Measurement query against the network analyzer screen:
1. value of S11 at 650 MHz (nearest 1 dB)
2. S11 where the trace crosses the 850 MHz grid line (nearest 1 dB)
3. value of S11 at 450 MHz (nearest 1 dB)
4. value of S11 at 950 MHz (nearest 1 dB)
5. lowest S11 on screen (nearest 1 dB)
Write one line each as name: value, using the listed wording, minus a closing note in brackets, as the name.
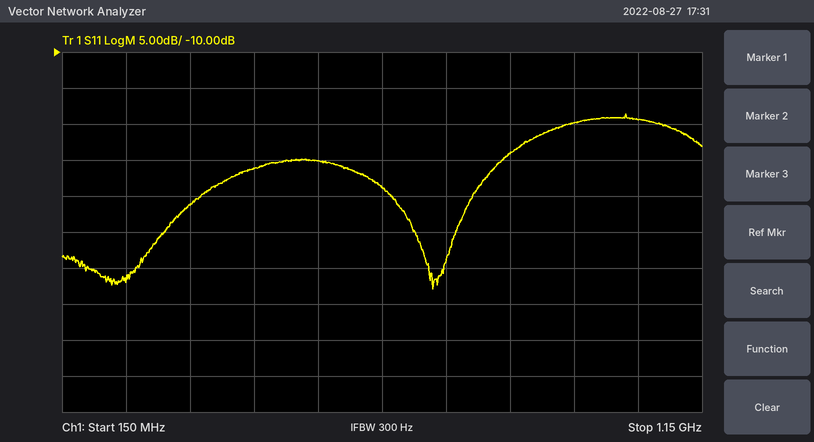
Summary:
value of S11 at 650 MHz: -29 dB
S11 where the trace crosses the 850 MHz grid line: -24 dB
value of S11 at 450 MHz: -26 dB
value of S11 at 950 MHz: -20 dB
lowest S11 on screen: -43 dB
